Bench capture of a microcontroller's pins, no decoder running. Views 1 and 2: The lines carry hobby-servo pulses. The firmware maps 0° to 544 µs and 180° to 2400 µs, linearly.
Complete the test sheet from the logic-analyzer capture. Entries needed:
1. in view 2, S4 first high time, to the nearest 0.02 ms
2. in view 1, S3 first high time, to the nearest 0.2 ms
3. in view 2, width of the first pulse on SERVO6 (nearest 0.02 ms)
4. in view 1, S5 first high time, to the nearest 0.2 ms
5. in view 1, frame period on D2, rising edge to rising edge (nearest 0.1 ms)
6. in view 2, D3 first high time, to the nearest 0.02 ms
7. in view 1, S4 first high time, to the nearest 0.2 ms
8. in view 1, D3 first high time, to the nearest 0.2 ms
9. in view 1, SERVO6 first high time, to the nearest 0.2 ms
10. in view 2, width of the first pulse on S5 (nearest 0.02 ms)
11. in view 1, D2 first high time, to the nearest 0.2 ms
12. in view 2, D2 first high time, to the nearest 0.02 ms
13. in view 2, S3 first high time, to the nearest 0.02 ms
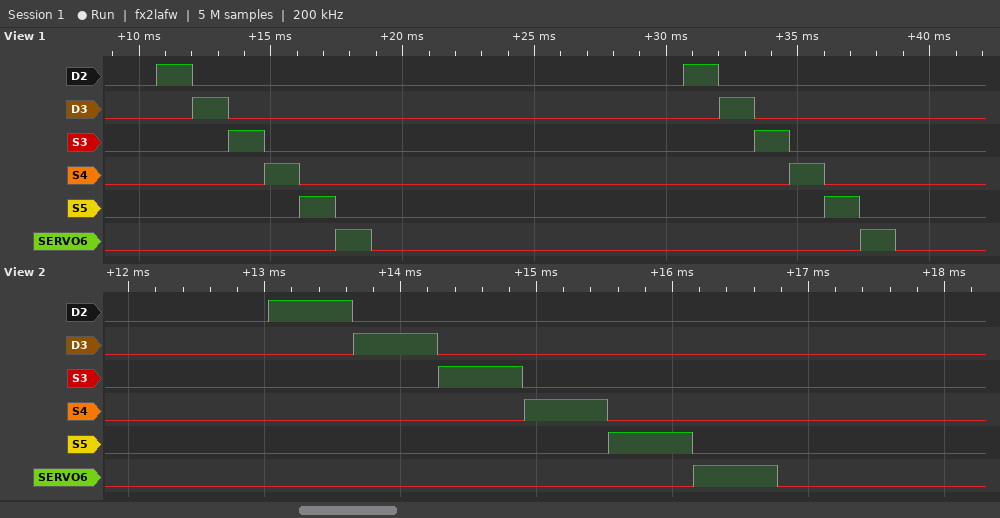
0.62 ms
1.4 ms
0.62 ms
1.4 ms
20.0 ms
0.62 ms
1.4 ms
1.4 ms
1.4 ms
0.62 ms
1.4 ms
0.62 ms
0.62 ms
